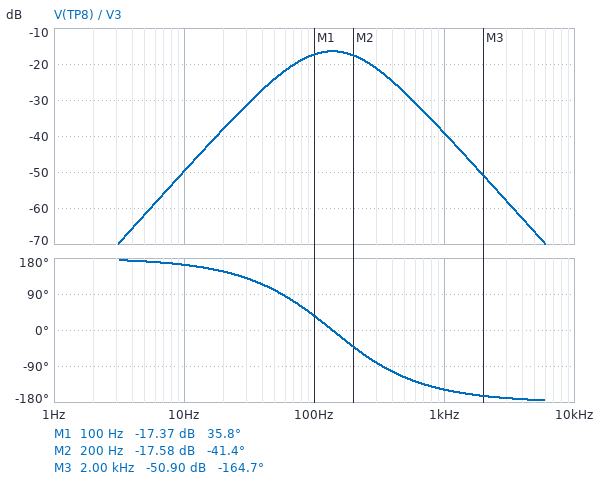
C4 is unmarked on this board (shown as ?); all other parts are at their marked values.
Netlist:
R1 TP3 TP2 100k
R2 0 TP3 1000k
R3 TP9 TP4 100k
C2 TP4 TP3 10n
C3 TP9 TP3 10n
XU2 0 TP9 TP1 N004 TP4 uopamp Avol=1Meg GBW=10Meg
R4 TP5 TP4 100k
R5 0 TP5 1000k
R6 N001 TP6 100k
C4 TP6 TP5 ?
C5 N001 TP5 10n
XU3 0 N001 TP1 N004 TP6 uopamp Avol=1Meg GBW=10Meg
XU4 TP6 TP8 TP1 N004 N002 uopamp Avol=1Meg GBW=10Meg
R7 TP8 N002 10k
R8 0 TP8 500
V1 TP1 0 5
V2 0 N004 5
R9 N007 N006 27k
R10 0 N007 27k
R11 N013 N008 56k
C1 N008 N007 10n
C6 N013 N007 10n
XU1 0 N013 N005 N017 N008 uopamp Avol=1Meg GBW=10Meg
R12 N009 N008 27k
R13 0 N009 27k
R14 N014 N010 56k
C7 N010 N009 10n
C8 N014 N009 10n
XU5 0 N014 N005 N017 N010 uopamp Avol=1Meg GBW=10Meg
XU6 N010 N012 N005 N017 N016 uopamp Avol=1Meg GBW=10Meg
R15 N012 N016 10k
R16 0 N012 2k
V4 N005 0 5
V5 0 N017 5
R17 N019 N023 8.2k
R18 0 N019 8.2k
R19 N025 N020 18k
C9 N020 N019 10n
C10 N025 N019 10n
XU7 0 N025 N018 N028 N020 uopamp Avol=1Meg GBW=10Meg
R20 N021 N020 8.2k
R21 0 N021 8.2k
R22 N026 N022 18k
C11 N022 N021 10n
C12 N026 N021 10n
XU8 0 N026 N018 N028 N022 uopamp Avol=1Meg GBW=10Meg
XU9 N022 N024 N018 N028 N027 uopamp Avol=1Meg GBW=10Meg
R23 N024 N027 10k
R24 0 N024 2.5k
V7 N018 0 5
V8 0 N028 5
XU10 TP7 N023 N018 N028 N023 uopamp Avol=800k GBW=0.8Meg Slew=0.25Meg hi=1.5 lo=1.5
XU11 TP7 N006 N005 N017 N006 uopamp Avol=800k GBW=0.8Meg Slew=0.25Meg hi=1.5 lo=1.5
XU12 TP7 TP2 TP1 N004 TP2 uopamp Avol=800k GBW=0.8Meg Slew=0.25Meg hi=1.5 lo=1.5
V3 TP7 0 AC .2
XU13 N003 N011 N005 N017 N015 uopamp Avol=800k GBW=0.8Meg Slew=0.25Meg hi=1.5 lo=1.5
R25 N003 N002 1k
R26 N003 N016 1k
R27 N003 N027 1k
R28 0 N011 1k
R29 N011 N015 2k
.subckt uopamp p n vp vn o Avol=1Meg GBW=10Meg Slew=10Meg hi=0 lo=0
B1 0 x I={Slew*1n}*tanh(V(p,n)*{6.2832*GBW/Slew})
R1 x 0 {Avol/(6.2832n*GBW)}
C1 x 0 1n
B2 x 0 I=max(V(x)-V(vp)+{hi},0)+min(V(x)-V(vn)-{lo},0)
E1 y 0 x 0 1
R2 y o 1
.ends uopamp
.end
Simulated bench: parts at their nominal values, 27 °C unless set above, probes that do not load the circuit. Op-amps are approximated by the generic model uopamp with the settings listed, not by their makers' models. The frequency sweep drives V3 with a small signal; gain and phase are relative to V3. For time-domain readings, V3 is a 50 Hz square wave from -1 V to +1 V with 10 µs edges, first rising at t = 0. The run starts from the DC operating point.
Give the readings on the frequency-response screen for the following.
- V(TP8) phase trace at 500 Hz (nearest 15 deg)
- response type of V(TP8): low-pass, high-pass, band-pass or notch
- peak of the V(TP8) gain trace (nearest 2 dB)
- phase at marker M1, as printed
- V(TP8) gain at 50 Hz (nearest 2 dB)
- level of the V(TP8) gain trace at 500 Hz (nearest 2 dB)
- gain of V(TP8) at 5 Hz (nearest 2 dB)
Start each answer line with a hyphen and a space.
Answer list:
- -120 deg
- band-pass
- -16 dB
- 35.8 deg
- -24 dB
- -28 dB
- -62 dB
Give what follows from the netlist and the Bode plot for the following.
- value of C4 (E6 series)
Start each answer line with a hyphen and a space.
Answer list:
- 22 nF
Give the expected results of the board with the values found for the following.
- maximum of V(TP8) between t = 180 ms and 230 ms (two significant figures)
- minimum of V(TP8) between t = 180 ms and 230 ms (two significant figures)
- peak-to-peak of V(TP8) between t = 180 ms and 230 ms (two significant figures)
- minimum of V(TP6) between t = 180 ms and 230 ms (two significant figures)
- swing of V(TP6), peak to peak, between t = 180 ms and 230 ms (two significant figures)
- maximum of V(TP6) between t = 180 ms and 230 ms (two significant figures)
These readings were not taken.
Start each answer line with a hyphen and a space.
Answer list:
- 170 mV
- -170 mV
- 330 mV
- -170 mV
- 330 mV
- 170 mV
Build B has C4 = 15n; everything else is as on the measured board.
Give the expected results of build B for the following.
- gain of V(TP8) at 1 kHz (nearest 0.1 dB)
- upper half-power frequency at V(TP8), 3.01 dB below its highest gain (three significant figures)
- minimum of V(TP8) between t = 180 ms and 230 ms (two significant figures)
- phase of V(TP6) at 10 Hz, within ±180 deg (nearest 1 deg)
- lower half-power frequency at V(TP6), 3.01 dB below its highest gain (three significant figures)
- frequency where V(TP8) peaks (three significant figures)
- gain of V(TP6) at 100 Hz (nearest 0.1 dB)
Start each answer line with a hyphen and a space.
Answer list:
- -35.8 dB
- 272 Hz
- -210 mV
- 165 deg
- 83.8 Hz
- 151 Hz
- -15.6 dB
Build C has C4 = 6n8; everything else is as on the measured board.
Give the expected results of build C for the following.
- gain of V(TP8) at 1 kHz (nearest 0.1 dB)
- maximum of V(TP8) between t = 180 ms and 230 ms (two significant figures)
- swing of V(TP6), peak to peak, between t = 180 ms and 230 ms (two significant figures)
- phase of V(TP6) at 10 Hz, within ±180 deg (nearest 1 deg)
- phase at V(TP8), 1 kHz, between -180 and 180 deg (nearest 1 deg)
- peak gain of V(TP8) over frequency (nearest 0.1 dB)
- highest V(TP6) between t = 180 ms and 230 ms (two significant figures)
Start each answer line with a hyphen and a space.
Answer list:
- -29.1 dB
- 240 mV
- 600 mV
- 168 deg
- -140 deg
- -10.6 dB
- 300 mV
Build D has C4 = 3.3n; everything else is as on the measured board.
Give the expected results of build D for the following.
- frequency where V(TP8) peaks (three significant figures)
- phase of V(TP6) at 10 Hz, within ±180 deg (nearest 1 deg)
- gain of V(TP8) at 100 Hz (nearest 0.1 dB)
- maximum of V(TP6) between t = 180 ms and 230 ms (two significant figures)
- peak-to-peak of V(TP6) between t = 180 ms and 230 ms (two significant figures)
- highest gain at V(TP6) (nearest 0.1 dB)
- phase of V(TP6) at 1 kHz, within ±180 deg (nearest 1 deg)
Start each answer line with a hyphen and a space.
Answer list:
- 212 Hz
- 169 deg
- -13.4 dB
- 380 mV
- 760 mV
- -9.1 dB
- -127 deg
